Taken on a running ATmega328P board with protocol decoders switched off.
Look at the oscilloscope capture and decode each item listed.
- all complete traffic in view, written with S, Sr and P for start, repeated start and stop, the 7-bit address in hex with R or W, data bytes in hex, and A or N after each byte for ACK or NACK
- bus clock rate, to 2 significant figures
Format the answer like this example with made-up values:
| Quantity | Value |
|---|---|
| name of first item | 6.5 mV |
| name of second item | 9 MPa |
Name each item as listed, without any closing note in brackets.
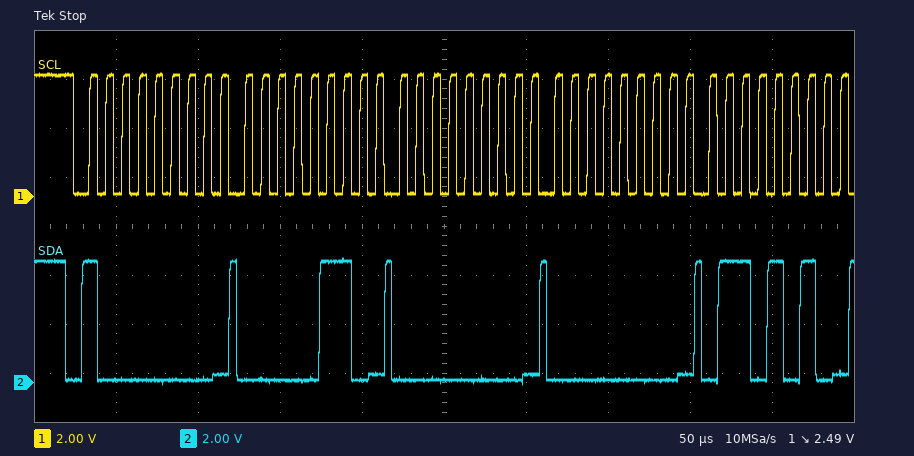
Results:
| Quantity | Value |
|---|---|
| all complete traffic in view, written with S, Sr and P for start, repeated start and stop, the 7-bit address in hex with R or W, data bytes in hex, and A or N after each byte for ACK or NACK | S 40W A 06 A 00 A 00 A 6A A |
| bus clock rate, to 2 significant figures | 100 kHz |
